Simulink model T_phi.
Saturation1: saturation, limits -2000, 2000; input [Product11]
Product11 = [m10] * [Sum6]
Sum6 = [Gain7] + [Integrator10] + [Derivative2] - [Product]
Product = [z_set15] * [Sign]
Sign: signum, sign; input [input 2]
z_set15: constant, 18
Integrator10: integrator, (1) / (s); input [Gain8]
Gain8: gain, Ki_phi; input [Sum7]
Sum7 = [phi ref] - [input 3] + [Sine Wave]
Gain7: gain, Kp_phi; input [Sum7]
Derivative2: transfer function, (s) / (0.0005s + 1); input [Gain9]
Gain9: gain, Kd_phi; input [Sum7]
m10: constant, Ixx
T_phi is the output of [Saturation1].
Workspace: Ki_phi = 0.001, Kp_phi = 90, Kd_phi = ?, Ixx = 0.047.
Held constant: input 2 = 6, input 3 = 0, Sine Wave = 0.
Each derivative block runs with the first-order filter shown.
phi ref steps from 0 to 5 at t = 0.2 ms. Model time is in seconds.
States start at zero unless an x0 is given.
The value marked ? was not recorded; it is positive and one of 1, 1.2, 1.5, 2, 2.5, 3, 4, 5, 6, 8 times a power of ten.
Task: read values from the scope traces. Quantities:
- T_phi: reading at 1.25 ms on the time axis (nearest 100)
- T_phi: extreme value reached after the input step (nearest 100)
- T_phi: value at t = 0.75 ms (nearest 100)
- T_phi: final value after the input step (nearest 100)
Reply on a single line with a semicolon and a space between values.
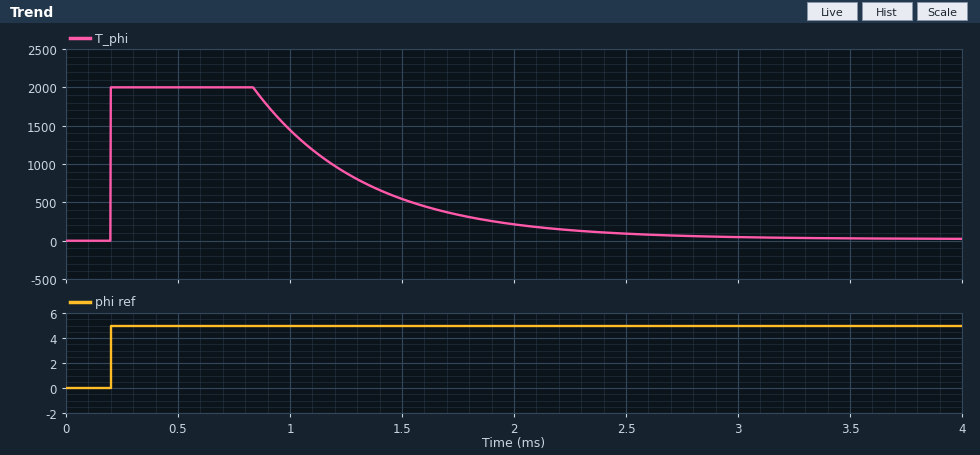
900; 2000; 2000; 0
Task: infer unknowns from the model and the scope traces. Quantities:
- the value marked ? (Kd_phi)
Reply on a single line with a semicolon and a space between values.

15
